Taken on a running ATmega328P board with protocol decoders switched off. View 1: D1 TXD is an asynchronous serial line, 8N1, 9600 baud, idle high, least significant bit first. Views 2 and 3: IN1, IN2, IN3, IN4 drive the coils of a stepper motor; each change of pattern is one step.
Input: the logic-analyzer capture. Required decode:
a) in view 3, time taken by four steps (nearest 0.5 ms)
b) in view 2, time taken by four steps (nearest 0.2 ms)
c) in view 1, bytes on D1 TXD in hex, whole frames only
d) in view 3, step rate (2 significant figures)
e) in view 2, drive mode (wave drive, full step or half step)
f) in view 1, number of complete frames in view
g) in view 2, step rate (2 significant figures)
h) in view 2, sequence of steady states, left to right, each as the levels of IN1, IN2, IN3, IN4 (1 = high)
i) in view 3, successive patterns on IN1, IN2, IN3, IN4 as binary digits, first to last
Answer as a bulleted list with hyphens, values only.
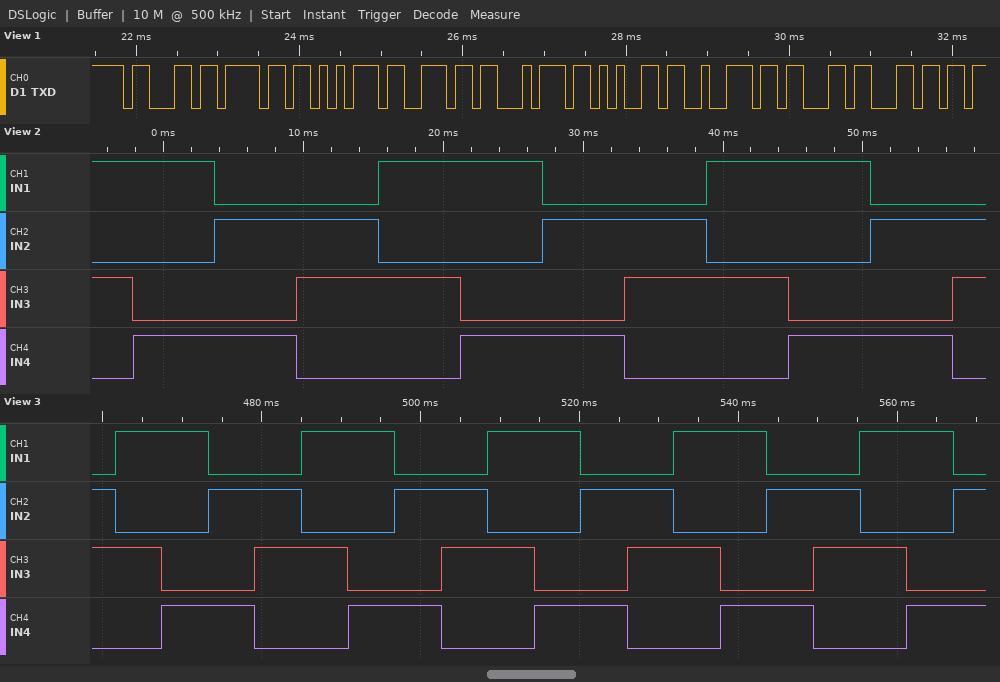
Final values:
- 23.5 ms
- 23.4 ms
- 63 6F 75 6E 74 65 72 63 6C
- 170 steps/s
- full step
- 9
- 170 steps/s
- 1010 1001 0101 0110 1010 1001 0101 0110 1010 1001 0101 0110
- 0110 1010 1001 0101 0110 1010 1001 0101 0110 1010 1001 0101 0110 1010 1001 0101 0110 1010 1001 0101
